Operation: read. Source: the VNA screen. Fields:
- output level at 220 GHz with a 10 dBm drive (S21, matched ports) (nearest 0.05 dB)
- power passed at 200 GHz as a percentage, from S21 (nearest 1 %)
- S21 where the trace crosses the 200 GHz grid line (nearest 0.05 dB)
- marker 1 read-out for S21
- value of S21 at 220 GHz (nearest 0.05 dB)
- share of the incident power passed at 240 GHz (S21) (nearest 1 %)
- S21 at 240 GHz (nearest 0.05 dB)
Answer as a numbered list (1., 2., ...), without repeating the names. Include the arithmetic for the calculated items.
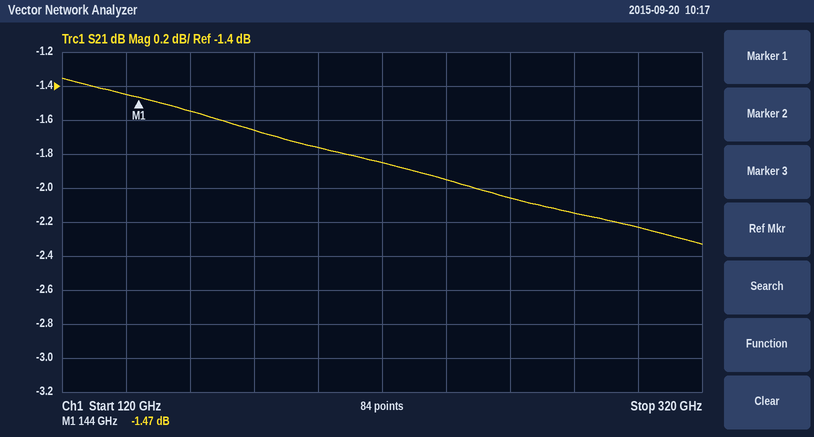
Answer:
1. 10 dBm + (-1.85 dB) = 8.15 dBm
2. 10^(-1.75/10) ≈ 67 %
3. -1.75 dB
4. -1.47 dB
5. -1.85 dB
6. 10^(-1.95/10) ≈ 64 %
7. -1.95 dB
